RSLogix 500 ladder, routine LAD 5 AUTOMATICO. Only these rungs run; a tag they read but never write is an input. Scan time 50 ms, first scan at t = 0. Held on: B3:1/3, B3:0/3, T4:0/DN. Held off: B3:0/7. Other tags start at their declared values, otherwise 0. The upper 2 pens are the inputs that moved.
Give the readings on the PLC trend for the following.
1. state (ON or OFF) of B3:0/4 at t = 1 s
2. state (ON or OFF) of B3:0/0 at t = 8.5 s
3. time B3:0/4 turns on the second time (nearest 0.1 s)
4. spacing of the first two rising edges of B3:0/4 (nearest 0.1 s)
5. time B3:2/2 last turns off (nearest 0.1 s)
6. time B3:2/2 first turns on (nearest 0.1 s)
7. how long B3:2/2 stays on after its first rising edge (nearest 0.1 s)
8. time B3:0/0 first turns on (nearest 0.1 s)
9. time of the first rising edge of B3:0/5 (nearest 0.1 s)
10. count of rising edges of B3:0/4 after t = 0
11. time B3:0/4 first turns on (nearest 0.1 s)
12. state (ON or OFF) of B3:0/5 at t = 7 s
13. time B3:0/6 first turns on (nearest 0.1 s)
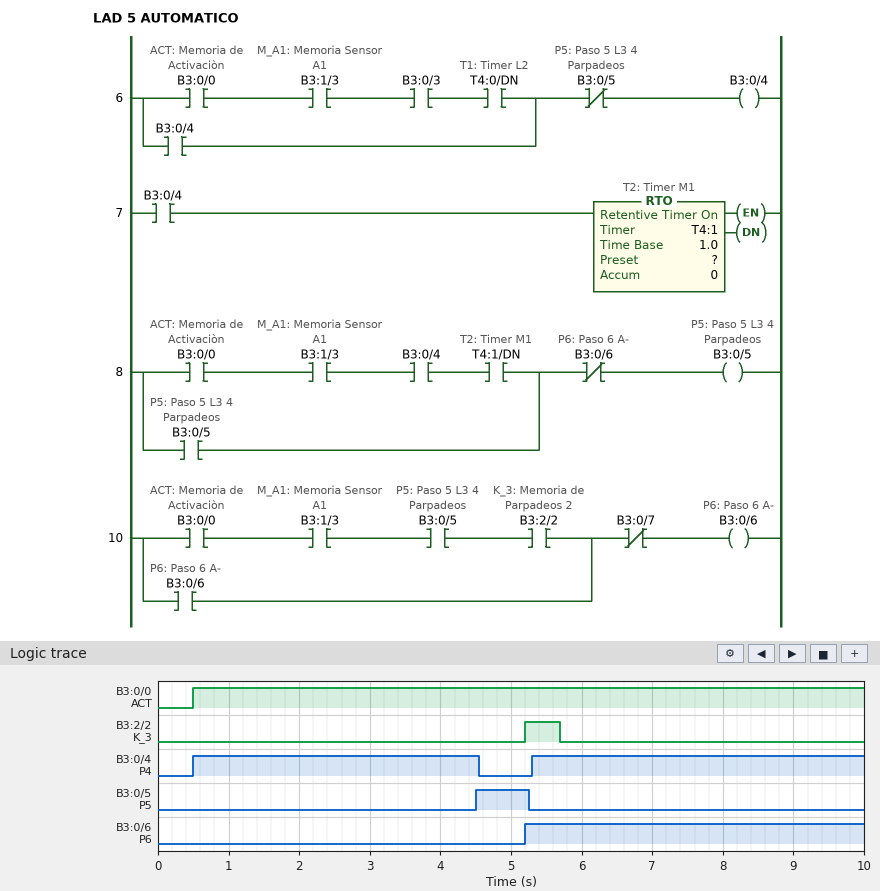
ON
ON
5.3 s
4.8 s
5.7 s
5.2 s
0.5 s
0.5 s
4.5 s
2
0.5 s
OFF
5.2 s
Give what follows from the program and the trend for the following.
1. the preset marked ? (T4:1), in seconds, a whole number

4 s
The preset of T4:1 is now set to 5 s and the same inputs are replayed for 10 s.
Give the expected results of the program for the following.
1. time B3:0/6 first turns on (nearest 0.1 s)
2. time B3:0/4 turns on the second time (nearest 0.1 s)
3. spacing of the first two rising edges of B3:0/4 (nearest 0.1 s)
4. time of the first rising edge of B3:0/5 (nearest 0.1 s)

5.5 s
5.6 s
5.1 s
5.5 s
